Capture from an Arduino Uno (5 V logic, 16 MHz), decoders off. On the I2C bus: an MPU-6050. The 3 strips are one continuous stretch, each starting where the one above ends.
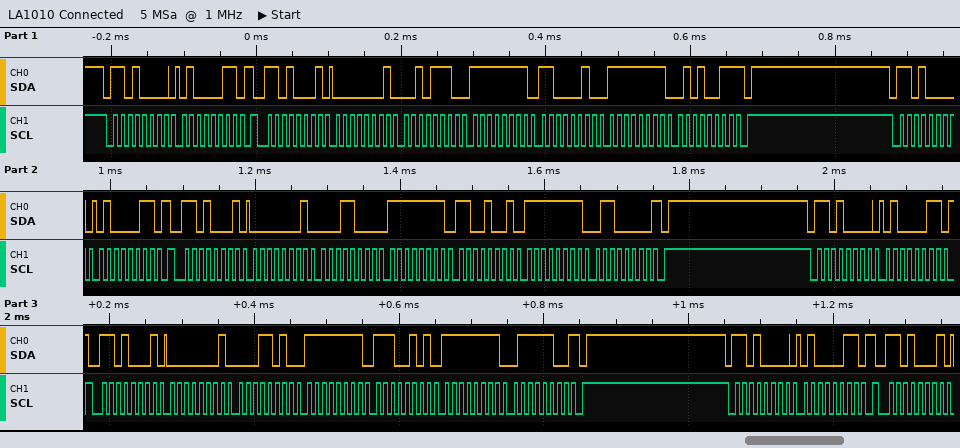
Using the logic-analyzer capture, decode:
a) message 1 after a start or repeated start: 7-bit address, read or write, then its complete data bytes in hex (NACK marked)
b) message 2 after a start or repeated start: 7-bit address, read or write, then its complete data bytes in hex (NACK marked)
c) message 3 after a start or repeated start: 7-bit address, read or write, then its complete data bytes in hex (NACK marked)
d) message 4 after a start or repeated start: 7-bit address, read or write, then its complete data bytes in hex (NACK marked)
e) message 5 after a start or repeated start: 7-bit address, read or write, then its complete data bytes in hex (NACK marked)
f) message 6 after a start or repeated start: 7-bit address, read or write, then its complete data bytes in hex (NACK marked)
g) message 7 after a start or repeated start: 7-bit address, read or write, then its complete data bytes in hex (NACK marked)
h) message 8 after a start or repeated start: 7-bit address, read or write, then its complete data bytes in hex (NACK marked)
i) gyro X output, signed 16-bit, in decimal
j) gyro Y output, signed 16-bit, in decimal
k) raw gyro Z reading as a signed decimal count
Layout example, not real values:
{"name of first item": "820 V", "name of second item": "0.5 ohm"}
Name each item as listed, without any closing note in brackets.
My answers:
{"message 1 after a start or repeated start: 7-bit address, read or write, then its complete data bytes in hex": "0x68 write: 43", "message 2 after a start or repeated start: 7-bit address, read or write, then its complete data bytes in hex": "0x68 read: 01 2E FF C2 FF 53 NACK", "message 3 after a start or repeated start: 7-bit address, read or write, then its complete data bytes in hex": "0x68 write: 43", "message 4 after a start or repeated start: 7-bit address, read or write, then its complete data bytes in hex": "0x68 read: 01 18 FF C9 FF 60 NACK", "message 5 after a start or repeated start: 7-bit address, read or write, then its complete data bytes in hex": "0x68 write: 43", "message 6 after a start or repeated start: 7-bit address, read or write, then its complete data bytes in hex": "0x68 read: 01 1A FF E5 FF 7C NACK", "message 7 after a start or repeated start: 7-bit address, read or write, then its complete data bytes in hex": "0x68 write: 43", "message 8 after a start or repeated start: 7-bit address, read or write, then its complete data bytes in hex": "0x68 read", "gyro X output, signed 16-bit, in decimal": "302", "gyro Y output, signed 16-bit, in decimal": "-62", "raw gyro Z reading as a signed decimal count": "-173"}
